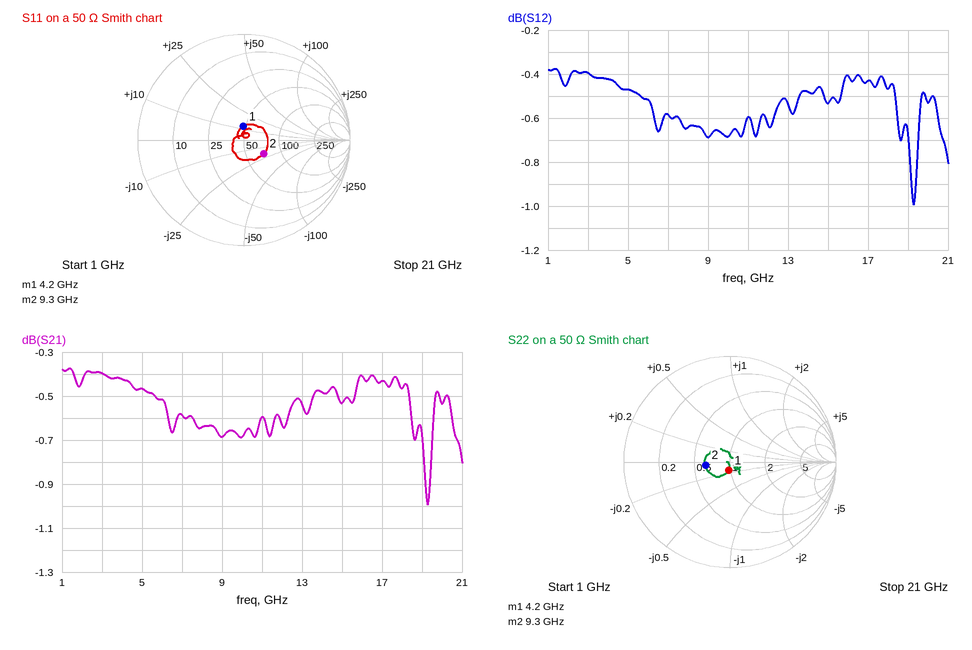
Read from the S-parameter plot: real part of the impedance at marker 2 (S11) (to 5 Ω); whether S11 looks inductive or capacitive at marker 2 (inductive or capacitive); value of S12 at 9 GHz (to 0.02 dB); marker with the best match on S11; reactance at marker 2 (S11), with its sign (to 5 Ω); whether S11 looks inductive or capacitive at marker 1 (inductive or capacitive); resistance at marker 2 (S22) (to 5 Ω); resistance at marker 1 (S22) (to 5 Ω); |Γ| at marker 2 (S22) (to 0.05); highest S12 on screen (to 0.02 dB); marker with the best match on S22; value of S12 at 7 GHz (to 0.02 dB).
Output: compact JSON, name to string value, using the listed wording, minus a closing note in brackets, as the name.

{"real part of the impedance at marker 2 (S11)": "70 Ω", "whether S11 looks inductive or capacitive at marker 2": "capacitive", "value of S12 at 9 GHz": "-0.68 dB", "marker with the best match on S11": "marker 1", "reactance at marker 2 (S11), with its sign": "-20 Ω", "whether S11 looks inductive or capacitive at marker 1": "inductive", "resistance at marker 2 (S22)": "30 Ω", "resistance at marker 1 (S22)": "50 Ω", "|Γ| at marker 2 (S22)": "0.25", "highest S12 on screen": "-0.38 dB", "marker with the best match on S22": "marker 1", "value of S12 at 7 GHz": "-0.58 dB"}
